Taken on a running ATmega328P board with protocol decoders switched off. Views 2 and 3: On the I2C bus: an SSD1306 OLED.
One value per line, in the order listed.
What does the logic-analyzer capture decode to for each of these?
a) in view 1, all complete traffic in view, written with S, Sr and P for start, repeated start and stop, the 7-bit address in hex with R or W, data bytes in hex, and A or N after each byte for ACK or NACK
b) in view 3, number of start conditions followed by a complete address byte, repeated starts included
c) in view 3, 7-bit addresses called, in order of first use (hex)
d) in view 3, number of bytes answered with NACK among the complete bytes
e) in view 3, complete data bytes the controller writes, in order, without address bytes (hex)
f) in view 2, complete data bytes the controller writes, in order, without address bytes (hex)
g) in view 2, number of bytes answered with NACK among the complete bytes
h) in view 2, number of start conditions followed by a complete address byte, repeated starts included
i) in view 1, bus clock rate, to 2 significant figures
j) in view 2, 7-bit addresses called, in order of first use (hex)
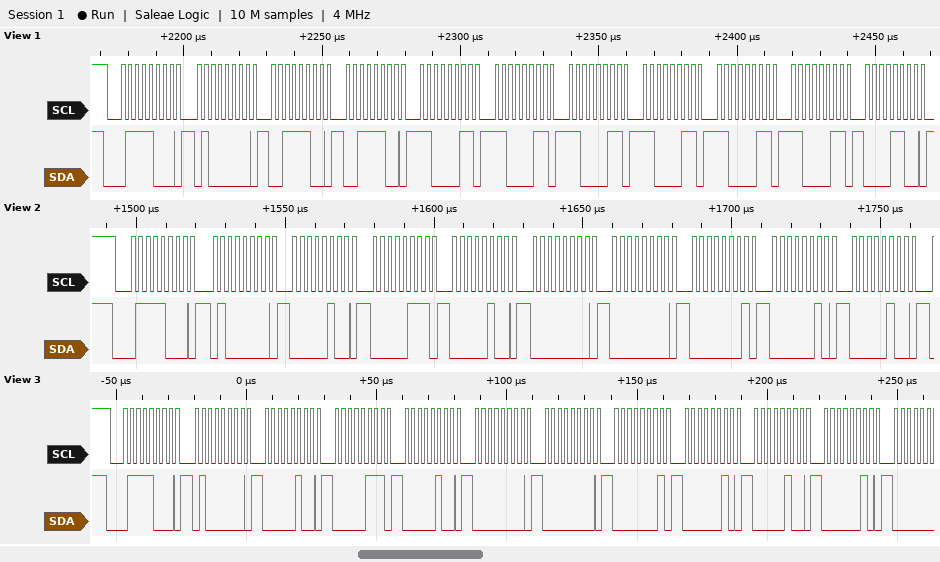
S 3CW A 40 A 3C A 3C A C3 A C3 A C3 A C3 A C3 A C3 A 0C A
1
0x3C
0
40 04 07 04 00 00 01 02 04 02
40 04 07 04 00 00 01 02 04
0
1
400 kHz
0x3C
